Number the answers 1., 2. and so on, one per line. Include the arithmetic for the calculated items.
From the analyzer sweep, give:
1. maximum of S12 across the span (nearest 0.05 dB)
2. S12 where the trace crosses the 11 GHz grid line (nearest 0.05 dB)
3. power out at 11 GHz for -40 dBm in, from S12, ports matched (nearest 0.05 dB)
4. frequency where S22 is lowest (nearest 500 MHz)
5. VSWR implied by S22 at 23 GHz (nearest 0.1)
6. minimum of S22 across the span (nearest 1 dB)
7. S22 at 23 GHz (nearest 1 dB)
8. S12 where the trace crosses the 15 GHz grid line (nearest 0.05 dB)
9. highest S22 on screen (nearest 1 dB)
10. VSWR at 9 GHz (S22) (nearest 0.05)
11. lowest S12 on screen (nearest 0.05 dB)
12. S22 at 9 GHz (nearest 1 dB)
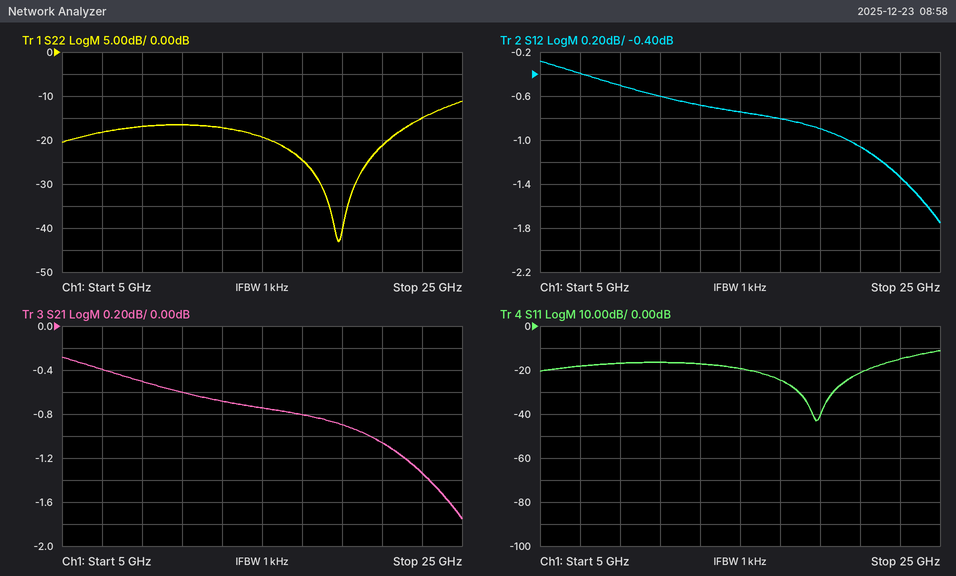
1. -0.30 dB
2. -0.60 dB
3. -40 dBm + (-0.60 dB) = -40.60 dBm
4. 19.0 GHz
5. |Γ| = 10^(-15/20) = 0.1778; VSWR = (1 + 0.1778)/(1 − 0.1778) ≈ 1.4
6. -43 dB
7. -15 dB
8. -0.75 dB
9. -11 dB
10. |Γ| = 10^(-17/20) = 0.1413; VSWR = (1 + 0.1413)/(1 − 0.1413) ≈ 1.33, so 1.35 to the nearest 0.05
11. -1.75 dB
12. -17 dB
